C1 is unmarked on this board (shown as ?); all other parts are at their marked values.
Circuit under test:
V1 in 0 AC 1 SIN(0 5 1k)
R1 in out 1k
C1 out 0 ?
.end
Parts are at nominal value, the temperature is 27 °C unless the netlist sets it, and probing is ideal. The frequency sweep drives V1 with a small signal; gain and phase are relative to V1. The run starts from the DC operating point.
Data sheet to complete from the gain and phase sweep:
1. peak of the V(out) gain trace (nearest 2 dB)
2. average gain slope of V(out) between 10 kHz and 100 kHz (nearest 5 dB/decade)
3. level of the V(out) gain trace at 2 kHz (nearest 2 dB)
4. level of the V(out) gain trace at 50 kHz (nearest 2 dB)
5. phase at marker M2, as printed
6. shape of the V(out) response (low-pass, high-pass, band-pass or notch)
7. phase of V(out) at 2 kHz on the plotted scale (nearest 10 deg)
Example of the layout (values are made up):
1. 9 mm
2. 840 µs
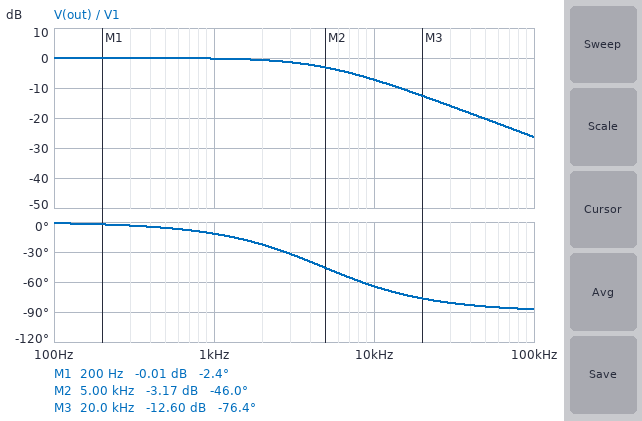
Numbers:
1. 0 dB
2. -20 dB/decade
3. 0 dB
4. -20 dB
5. -46.0 deg
6. low-pass
7. -20 deg
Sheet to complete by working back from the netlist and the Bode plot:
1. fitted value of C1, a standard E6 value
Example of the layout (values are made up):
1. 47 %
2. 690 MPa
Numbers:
1. 33 nF
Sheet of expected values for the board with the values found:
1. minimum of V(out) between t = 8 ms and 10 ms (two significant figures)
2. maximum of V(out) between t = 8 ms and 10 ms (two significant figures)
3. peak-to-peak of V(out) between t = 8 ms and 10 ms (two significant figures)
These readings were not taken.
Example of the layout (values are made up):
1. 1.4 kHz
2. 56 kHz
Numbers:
1. -4.9 V
2. 4.9 V
3. 9.8 V
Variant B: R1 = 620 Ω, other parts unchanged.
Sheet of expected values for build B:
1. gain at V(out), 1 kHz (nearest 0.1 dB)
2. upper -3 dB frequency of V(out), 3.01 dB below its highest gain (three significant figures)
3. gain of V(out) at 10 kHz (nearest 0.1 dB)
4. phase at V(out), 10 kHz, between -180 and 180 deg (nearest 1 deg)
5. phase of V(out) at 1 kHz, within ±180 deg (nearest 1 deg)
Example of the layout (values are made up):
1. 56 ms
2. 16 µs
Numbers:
1. -0.1 dB
2. 7.78 kHz
3. -4.2 dB
4. -52 deg
5. -7 deg
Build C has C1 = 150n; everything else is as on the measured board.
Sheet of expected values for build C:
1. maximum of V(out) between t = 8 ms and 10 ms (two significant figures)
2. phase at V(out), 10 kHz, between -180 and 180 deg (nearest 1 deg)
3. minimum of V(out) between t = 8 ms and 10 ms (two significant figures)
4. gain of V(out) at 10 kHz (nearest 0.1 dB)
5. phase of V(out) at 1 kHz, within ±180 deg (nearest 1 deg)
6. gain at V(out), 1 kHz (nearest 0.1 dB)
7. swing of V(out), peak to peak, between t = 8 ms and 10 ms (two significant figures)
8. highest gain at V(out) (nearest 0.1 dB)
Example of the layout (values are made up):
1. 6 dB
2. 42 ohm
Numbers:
1. 3.6 V
2. -84 deg
3. -3.6 V
4. -19.5 dB
5. -43 deg
6. -2.8 dB
7. 7.3 V
8. 0 dB
